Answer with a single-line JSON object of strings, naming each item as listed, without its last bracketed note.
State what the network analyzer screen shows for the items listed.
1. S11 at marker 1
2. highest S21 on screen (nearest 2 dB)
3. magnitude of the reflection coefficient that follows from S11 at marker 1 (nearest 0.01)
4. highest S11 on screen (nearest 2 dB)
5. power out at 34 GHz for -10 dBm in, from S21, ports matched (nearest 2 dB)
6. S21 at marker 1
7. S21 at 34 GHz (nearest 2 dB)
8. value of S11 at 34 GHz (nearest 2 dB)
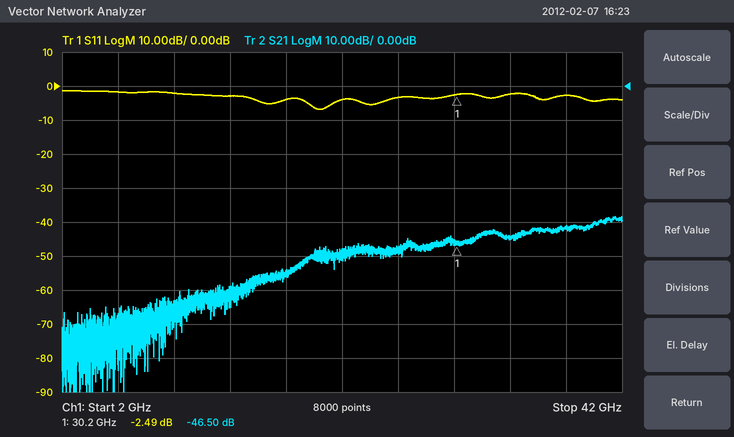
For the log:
{"S11 at marker 1": "-2.49 dB", "highest S21 on screen": "-38 dB", "magnitude of the reflection coefficient that follows from S11 at marker 1": "0.75", "highest S11 on screen": "-2 dB", "power out at 34 GHz for -10 dBm in, from S21, ports matched": "-54 dBm", "S21 at marker 1": "-46.50 dB", "S21 at 34 GHz": "-44 dB", "value of S11 at 34 GHz": "-2 dB"}
